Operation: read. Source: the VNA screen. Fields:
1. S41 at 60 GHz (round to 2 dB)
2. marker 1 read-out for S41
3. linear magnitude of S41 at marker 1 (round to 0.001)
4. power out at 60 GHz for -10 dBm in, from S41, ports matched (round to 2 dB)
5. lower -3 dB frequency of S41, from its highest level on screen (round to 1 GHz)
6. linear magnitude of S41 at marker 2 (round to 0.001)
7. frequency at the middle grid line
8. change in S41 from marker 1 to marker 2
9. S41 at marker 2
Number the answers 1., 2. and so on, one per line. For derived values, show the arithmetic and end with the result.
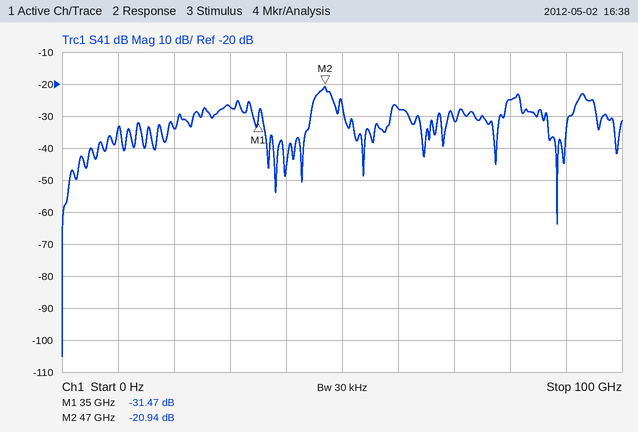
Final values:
1. -28 dB
2. -31.47 dB
3. 10^(-31.47/20) ≈ 0.027
4. -10 dBm + (-28 dB) = -38 dBm
5. 45 GHz
6. 10^(-20.94/20) ≈ 0.090
7. 50 GHz
8. -20.94 − (-31.47) = 10.53 dB
9. -20.94 dB
